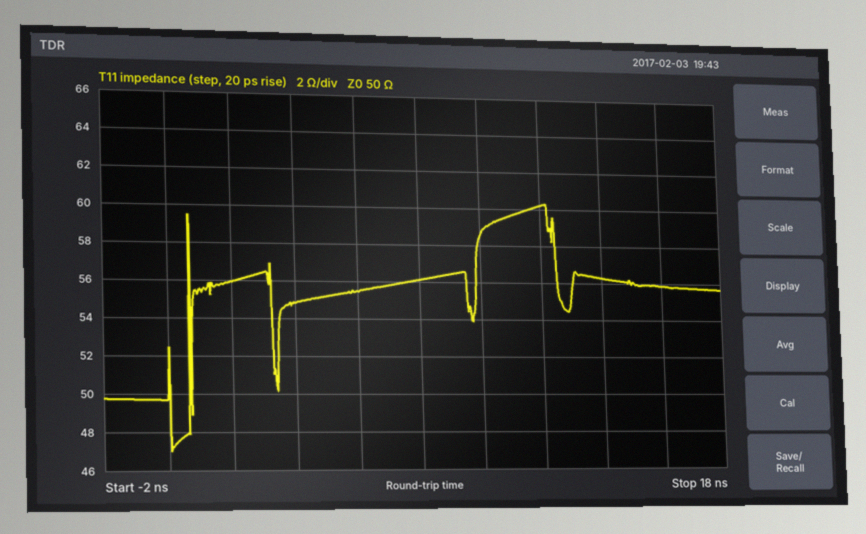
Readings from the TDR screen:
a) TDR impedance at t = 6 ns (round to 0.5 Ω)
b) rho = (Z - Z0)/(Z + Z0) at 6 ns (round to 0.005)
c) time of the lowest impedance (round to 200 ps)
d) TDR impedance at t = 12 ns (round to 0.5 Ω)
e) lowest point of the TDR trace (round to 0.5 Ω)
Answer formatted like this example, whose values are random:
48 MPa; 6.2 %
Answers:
55.5 Ω; +0.050; 0.0 ns; 60.0 Ω; 47.0 Ω
